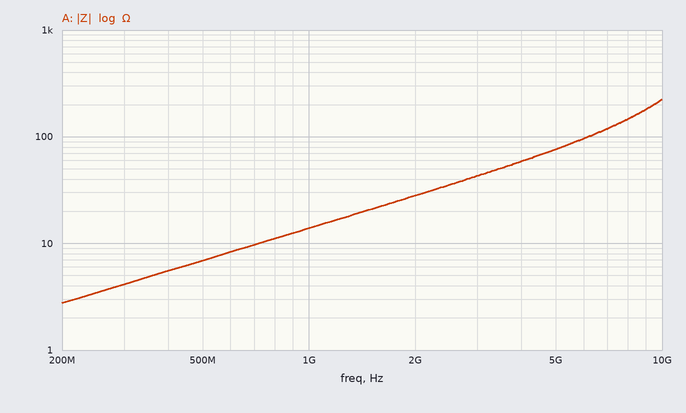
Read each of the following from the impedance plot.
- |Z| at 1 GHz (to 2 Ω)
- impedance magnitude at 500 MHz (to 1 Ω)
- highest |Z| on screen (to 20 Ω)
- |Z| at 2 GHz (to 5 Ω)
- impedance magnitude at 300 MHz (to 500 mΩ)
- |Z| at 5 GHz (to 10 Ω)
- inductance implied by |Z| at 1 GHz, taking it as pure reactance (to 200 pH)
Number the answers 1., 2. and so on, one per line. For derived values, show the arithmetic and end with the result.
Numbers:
1. 14 Ω
2. 7 Ω
3. 220 Ω
4. 30 Ω
5. 4.0 Ω
6. 80 Ω
7. L = 14 Ω/(2π × 1 GHz) ≈ 2.2 nH
